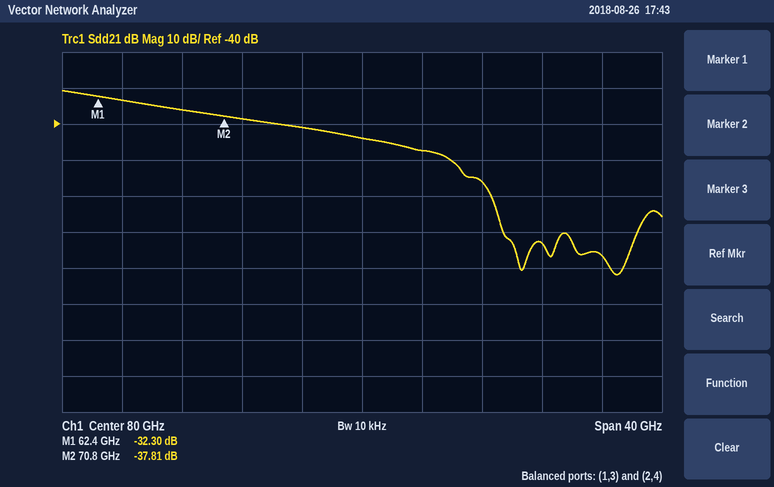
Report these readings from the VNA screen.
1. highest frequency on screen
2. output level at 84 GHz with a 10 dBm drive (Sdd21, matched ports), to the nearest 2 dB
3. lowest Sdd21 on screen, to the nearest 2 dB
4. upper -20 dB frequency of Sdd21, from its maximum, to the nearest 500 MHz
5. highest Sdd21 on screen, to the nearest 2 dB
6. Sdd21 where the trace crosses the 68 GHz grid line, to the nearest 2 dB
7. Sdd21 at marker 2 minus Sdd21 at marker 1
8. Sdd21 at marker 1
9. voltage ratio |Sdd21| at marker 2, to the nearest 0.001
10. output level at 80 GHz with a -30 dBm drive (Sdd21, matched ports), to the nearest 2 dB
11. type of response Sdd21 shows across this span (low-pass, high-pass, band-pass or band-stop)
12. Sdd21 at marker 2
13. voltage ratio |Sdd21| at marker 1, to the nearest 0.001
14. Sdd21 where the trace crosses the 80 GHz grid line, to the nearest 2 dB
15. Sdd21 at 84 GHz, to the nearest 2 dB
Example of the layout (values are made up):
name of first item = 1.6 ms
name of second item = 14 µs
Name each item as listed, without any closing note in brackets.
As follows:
highest frequency on screen = 100 GHz
output level at 84 GHz with a 10 dBm drive (Sdd21, matched ports), to the nearest 2 dB = -38 dBm
lowest Sdd21 on screen, to the nearest 2 dB = -82 dB
upper -20 dB frequency of Sdd21, from its maximum, to the nearest 500 MHz = 86.0 GHz
highest Sdd21 on screen, to the nearest 2 dB = -30 dB
Sdd21 where the trace crosses the 68 GHz grid line, to the nearest 2 dB = -36 dB
Sdd21 at marker 2 minus Sdd21 at marker 1 = -5.51 dB
Sdd21 at marker 1 = -32.30 dB
voltage ratio |Sdd21| at marker 2, to the nearest 0.001 = 0.013
output level at 80 GHz with a -30 dBm drive (Sdd21, matched ports), to the nearest 2 dB = -74 dBm
type of response Sdd21 shows across this span = low-pass
Sdd21 at marker 2 = -37.81 dB
voltage ratio |Sdd21| at marker 1, to the nearest 0.001 = 0.024
Sdd21 where the trace crosses the 80 GHz grid line, to the nearest 2 dB = -44 dB
Sdd21 at 84 GHz, to the nearest 2 dB = -48 dB
